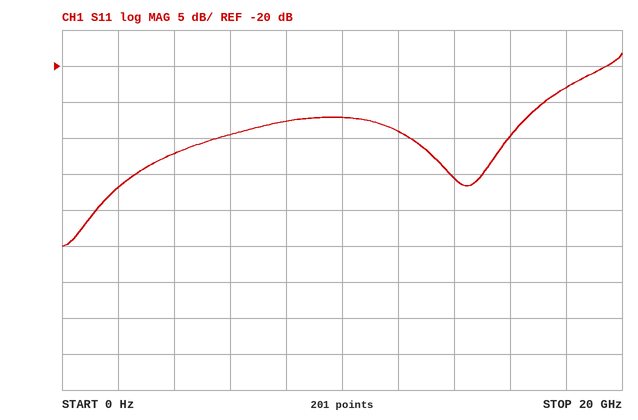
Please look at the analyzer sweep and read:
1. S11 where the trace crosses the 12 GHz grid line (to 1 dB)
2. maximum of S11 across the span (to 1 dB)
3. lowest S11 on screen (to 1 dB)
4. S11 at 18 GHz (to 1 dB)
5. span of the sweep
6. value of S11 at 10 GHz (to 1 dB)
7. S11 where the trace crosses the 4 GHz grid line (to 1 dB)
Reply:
-29 dB
-18 dB
-45 dB
-23 dB
20 GHz
-27 dB
-32 dB
